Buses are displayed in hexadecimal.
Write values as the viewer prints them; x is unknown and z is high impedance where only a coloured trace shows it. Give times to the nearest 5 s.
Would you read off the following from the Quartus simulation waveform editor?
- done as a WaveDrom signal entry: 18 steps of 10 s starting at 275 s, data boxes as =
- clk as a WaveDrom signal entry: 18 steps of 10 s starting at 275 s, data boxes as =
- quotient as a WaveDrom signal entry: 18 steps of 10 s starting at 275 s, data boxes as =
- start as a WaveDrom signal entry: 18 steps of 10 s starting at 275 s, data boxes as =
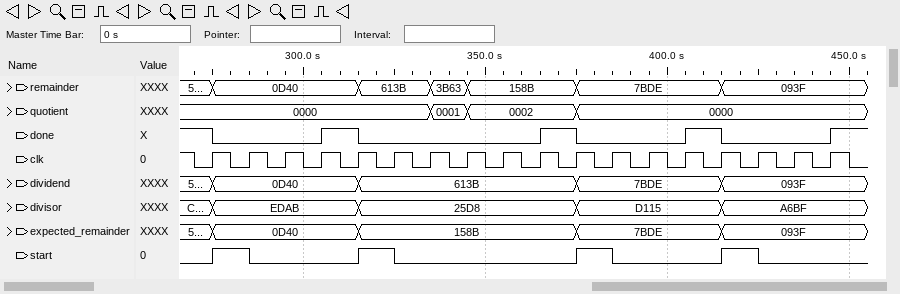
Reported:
{name: 'done', wave: '0..10....10..10..1'}
{name: 'clk', wave: 'p.................'}
{name: 'quotient', wave: '=.....==..=.......', data: '0000 0001 0002 0000'}
{name: 'start', wave: '10..10....10..10..'}
